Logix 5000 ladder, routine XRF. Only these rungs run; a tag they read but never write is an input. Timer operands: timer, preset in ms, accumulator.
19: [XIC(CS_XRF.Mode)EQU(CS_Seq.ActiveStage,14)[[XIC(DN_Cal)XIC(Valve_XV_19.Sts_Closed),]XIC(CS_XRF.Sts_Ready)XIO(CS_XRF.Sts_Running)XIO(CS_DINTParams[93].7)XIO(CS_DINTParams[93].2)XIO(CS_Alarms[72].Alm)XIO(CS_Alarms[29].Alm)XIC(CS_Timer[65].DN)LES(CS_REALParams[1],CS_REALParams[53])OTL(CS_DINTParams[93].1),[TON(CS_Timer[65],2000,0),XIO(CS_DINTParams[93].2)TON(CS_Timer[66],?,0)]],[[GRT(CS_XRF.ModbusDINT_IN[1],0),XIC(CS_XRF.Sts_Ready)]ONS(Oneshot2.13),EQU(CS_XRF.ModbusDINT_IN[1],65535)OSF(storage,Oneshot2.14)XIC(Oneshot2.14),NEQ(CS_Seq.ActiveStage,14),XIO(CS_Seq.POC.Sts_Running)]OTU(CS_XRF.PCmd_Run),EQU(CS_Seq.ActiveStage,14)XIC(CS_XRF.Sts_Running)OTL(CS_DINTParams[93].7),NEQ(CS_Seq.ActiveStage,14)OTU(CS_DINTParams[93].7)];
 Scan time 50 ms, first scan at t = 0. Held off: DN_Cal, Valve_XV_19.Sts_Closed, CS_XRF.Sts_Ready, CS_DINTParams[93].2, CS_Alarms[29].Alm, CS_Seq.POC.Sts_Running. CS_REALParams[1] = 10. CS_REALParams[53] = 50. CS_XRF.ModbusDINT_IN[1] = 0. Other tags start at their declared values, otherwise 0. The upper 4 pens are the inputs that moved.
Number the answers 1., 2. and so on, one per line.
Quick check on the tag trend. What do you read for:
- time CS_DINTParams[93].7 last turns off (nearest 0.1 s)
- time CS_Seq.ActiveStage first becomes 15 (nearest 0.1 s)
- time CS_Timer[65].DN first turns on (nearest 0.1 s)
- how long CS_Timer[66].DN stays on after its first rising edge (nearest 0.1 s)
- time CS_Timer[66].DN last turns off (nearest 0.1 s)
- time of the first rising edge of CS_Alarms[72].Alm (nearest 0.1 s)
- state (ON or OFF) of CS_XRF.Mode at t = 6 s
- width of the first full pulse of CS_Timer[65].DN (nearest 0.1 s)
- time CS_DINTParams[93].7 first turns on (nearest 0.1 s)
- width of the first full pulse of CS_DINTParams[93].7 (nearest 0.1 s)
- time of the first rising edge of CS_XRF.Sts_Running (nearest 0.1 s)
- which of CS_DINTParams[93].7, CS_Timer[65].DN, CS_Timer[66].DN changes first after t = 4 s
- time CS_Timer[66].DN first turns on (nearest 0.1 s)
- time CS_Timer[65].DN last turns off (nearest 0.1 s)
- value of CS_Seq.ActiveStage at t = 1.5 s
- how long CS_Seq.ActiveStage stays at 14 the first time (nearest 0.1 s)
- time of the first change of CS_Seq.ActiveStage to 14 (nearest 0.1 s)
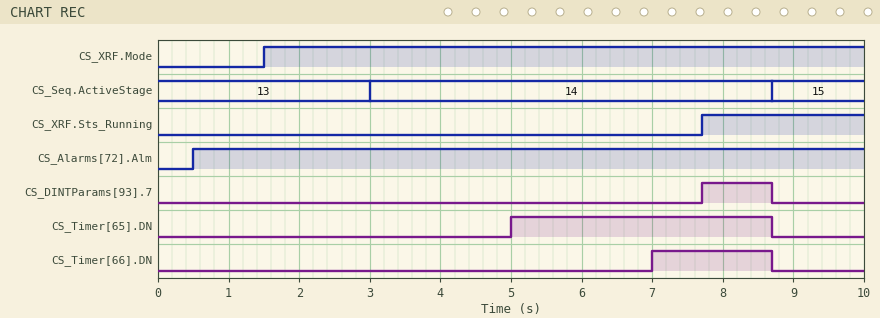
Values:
1. 8.7 s
2. 8.7 s
3. 5.0 s
4. 1.7 s
5. 8.7 s
6. 0.5 s
7. ON
8. 3.7 s
9. 7.7 s
10. 1.0 s
11. 7.7 s
12. CS_Timer[65].DN
13. 7.0 s
14. 8.7 s
15. 13
16. 5.7 s
17. 3.0 s
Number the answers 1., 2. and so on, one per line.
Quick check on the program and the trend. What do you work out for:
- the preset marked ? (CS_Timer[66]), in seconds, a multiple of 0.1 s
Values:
1. 4.0 s
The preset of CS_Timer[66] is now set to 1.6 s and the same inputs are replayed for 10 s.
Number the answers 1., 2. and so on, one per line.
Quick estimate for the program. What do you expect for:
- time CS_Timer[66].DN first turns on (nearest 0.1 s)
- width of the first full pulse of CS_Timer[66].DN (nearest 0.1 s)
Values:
1. 4.6 s
2. 4.1 s
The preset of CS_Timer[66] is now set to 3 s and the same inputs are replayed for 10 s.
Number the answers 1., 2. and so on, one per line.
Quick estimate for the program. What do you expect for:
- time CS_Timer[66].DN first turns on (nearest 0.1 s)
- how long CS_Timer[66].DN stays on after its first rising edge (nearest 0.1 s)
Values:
1. 6.0 s
2. 2.7 s
